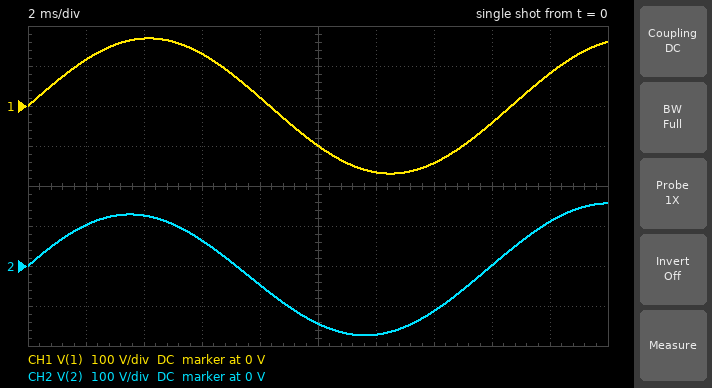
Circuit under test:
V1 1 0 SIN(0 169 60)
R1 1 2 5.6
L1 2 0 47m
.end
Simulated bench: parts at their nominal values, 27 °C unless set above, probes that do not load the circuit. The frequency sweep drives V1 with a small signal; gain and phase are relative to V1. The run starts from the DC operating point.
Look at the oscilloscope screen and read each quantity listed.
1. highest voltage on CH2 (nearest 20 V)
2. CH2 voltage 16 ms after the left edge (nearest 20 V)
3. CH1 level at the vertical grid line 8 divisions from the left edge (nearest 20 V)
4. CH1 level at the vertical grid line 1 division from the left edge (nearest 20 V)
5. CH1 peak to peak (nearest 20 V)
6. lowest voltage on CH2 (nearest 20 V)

160 V
0 V
-40 V
120 V
340 V
-180 V
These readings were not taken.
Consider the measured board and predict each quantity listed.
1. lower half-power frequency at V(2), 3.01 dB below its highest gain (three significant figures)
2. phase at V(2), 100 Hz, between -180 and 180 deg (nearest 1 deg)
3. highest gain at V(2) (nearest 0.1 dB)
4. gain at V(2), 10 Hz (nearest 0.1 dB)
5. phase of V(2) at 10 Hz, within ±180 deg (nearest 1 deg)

19.0 Hz
11 deg
0 dB
-6.6 dB
62 deg
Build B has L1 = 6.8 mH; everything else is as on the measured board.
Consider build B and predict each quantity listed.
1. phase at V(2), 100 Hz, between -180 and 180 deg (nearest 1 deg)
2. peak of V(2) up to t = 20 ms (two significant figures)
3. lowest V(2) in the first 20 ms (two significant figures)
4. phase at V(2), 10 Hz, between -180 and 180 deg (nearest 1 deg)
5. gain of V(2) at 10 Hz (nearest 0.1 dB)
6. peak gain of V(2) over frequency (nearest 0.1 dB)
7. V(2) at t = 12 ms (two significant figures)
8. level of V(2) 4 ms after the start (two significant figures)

53 deg
70 V
-70 V
86 deg
-22.4 dB
0 dB
-41 V
31 V
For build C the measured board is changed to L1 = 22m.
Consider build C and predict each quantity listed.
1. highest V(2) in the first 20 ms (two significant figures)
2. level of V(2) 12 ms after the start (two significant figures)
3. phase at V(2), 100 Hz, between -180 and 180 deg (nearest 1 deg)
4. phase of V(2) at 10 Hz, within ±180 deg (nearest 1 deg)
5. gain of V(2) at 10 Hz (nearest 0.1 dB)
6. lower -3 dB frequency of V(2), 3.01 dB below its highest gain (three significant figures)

140 V
-130 V
22 deg
76 deg
-12.4 dB
40.5 Hz
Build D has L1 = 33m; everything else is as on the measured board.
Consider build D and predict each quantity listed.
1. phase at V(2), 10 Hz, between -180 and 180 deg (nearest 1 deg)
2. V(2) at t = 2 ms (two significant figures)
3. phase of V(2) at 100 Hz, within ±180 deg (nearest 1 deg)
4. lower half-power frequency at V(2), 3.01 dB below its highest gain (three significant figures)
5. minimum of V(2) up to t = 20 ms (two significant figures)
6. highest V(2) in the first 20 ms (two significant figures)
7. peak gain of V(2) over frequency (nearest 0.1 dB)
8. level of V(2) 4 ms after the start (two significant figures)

70 deg
97 V
15 deg
27.0 Hz
-160 V
150 V
0 dB
110 V
